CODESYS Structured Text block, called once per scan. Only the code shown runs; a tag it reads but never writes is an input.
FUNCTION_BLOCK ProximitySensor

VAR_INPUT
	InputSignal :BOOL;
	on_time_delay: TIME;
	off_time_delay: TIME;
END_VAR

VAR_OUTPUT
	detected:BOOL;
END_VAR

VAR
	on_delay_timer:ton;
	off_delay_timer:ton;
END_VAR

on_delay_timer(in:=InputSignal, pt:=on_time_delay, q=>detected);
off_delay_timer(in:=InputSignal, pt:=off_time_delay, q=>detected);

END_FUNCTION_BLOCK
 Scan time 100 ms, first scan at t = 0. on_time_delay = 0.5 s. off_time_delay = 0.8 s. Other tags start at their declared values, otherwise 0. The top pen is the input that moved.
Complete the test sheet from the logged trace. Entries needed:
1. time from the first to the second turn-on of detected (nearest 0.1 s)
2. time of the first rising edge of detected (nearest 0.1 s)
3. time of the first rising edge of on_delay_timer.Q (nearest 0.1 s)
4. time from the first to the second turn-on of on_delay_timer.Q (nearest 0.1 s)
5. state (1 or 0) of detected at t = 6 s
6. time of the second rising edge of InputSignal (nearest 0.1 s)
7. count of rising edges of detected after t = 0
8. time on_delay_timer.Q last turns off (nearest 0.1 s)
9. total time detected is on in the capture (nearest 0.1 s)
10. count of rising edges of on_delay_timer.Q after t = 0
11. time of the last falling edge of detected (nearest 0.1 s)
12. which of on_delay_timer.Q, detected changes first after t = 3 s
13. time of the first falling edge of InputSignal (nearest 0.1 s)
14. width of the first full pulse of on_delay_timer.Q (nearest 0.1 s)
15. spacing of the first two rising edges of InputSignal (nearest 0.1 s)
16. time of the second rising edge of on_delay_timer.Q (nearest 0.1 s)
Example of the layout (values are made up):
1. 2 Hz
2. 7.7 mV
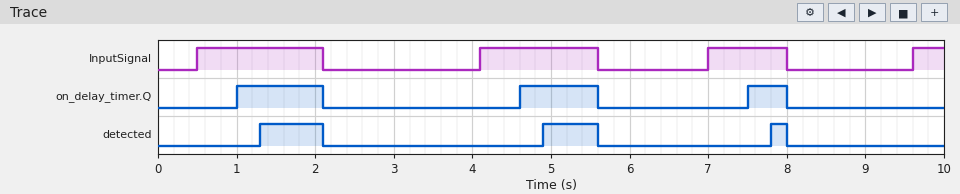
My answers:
1. 3.6 s
2. 1.3 s
3. 1.0 s
4. 3.6 s
5. 0
6. 4.1 s
7. 3
8. 8.0 s
9. 1.7 s
10. 3
11. 8.0 s
12. on_delay_timer.Q
13. 2.1 s
14. 1.1 s
15. 3.6 s
16. 4.6 s
